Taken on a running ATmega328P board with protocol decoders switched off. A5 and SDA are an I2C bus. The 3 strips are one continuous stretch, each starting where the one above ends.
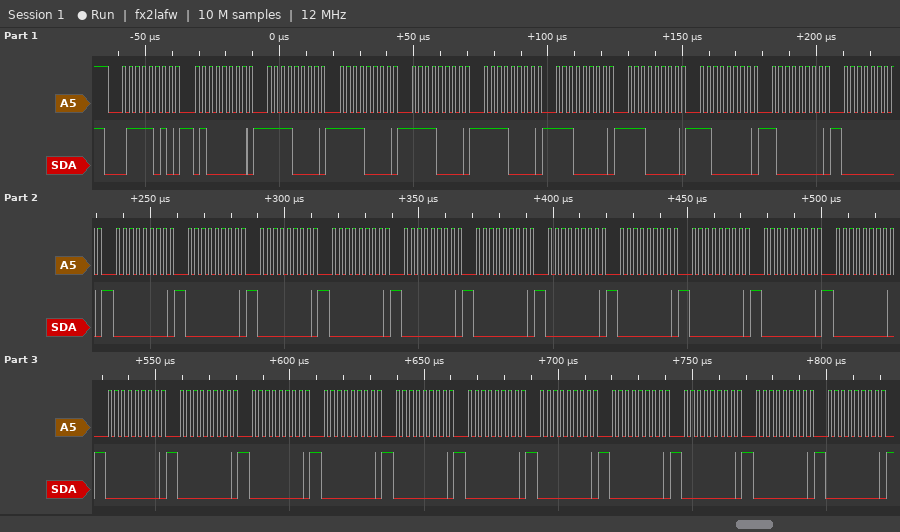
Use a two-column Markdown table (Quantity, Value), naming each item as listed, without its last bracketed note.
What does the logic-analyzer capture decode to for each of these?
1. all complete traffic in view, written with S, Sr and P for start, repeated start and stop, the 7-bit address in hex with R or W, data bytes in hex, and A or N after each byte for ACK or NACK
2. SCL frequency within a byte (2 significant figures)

| Quantity | Value |
|---|---|
| all complete traffic in view, written with S, Sr and P for start, repeated start and stop, the 7-bit address in hex with R or W, data bytes in hex, and A or N after each byte for ACK or NACK | S 3DW A 40 A F0 A F0 A F0 A F0 A E0 A E0 A C0 A 80 A 00 A 00 A 00 A 00 A 00 A 00 A 00 A 00 A 00 A 00 A 00 A 00 A 00 A 00 A 00 A 00 A 00 A 00 A 00 A 00 A 00 A 00 A 00 A |
| SCL frequency within a byte | 400 kHz |
